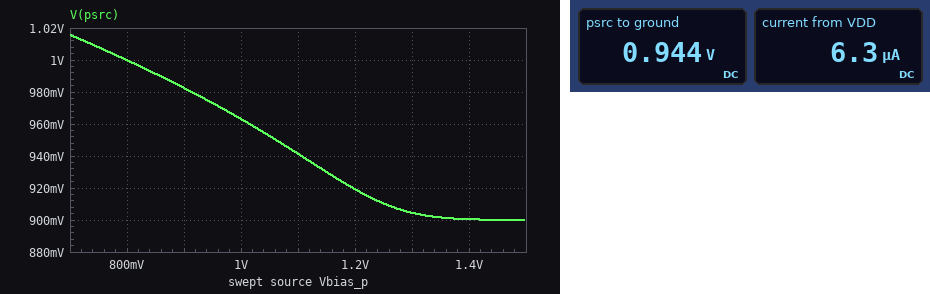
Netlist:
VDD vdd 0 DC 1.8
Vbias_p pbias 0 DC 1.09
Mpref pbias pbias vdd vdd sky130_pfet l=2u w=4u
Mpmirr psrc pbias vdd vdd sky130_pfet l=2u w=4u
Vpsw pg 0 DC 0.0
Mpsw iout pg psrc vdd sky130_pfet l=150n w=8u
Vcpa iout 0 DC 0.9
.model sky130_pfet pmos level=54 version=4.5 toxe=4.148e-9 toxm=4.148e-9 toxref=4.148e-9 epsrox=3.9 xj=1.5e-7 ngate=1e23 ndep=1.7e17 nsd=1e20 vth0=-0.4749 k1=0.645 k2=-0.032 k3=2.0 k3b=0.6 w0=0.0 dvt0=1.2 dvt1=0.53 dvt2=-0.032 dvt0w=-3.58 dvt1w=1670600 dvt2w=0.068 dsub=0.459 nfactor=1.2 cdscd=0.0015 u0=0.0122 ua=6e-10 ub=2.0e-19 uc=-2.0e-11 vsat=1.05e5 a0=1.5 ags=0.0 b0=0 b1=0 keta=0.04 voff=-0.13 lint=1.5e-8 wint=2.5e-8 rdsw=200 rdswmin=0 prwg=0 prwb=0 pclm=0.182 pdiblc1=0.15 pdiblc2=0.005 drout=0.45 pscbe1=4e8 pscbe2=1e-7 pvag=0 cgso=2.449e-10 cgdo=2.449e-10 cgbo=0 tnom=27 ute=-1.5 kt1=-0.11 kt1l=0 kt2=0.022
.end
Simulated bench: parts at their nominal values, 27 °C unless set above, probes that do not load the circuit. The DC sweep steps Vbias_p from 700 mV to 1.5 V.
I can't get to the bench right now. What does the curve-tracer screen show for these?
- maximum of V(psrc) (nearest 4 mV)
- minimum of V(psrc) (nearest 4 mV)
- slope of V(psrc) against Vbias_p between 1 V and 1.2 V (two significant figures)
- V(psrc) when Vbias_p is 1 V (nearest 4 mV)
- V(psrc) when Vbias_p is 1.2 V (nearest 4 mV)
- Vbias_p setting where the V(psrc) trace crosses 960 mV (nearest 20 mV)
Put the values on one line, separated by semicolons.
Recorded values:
1.016 V; 900 mV; -0.22 V/V; 964 mV; 920 mV; 1.02 V
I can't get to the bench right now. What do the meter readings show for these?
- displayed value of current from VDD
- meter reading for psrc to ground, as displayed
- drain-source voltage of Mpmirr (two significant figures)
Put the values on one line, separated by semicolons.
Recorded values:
6.3 µA; 0.944 V; -860 mV
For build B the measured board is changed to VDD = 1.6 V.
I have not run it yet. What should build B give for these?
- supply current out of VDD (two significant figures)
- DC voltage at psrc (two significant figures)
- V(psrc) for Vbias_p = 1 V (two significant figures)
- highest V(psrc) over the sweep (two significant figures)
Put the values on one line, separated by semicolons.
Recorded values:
440 nA; 900 mV; 910 mV; 960 mV
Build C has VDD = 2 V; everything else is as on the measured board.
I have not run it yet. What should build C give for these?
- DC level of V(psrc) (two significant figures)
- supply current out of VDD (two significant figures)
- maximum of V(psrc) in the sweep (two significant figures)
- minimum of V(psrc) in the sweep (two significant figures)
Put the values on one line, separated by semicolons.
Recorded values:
1.0 V; 21 µA; 1.1 V; 910 mV
